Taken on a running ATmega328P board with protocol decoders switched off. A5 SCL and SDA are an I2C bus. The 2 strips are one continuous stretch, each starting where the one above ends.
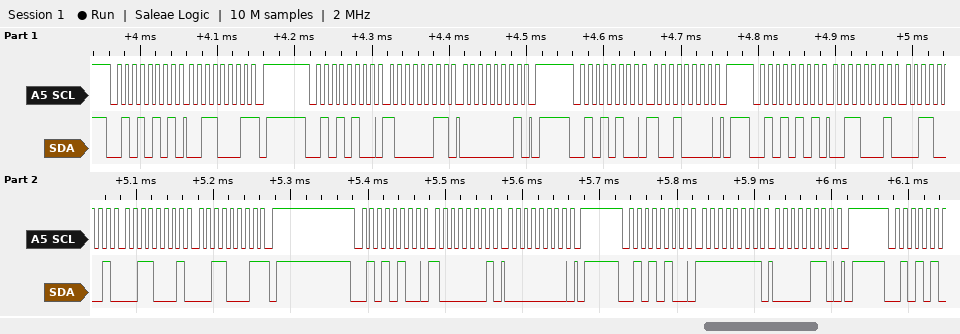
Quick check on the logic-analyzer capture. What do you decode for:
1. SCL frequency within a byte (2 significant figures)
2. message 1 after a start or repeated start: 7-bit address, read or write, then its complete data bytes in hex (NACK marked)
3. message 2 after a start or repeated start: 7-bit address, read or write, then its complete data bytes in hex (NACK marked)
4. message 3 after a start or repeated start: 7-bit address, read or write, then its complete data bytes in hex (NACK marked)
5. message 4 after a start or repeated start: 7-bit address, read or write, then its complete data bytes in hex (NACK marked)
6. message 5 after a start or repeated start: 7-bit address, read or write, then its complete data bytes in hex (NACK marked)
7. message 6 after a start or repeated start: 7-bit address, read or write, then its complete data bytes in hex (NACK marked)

100 kHz
0x2A read: 31 NACK
0x2A write: 83 01
0x2A write: 90
0x2A read: 31 31 31 31 NACK
0x2A write: 81 00
0x2A write: FF 06
